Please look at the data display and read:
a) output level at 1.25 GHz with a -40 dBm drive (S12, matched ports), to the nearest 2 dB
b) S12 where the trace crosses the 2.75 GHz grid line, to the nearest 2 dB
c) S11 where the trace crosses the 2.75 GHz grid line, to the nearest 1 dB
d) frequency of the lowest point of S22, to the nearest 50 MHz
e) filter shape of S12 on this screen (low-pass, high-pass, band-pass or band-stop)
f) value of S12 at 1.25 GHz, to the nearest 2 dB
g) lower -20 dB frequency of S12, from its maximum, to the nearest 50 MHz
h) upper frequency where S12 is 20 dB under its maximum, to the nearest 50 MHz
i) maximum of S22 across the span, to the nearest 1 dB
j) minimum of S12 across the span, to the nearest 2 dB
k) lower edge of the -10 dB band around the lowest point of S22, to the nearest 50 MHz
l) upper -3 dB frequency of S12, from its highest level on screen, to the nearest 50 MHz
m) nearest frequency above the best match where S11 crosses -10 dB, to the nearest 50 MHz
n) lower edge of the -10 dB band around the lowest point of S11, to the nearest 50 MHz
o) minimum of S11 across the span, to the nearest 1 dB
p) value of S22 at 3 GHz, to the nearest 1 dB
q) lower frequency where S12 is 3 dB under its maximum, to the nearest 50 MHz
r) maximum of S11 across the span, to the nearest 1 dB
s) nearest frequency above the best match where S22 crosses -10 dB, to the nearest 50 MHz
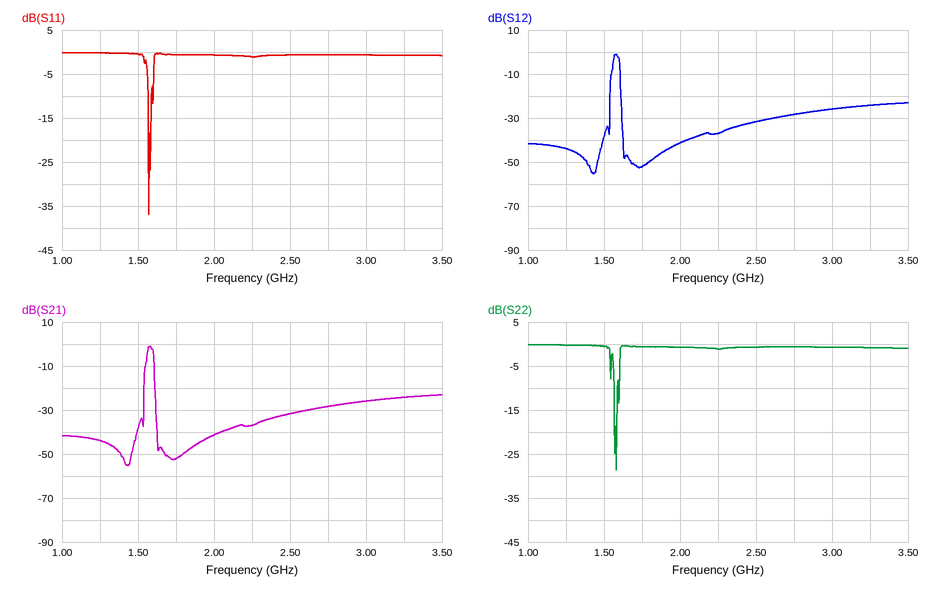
-84 dBm
-28 dB
-1 dB
1.60 GHz
band-pass
-44 dB
1.55 GHz
1.60 GHz
0 dB
-56 dB
1.55 GHz
1.60 GHz
1.60 GHz
1.55 GHz
-37 dB
-1 dB
1.55 GHz
0 dB
1.60 GHz
